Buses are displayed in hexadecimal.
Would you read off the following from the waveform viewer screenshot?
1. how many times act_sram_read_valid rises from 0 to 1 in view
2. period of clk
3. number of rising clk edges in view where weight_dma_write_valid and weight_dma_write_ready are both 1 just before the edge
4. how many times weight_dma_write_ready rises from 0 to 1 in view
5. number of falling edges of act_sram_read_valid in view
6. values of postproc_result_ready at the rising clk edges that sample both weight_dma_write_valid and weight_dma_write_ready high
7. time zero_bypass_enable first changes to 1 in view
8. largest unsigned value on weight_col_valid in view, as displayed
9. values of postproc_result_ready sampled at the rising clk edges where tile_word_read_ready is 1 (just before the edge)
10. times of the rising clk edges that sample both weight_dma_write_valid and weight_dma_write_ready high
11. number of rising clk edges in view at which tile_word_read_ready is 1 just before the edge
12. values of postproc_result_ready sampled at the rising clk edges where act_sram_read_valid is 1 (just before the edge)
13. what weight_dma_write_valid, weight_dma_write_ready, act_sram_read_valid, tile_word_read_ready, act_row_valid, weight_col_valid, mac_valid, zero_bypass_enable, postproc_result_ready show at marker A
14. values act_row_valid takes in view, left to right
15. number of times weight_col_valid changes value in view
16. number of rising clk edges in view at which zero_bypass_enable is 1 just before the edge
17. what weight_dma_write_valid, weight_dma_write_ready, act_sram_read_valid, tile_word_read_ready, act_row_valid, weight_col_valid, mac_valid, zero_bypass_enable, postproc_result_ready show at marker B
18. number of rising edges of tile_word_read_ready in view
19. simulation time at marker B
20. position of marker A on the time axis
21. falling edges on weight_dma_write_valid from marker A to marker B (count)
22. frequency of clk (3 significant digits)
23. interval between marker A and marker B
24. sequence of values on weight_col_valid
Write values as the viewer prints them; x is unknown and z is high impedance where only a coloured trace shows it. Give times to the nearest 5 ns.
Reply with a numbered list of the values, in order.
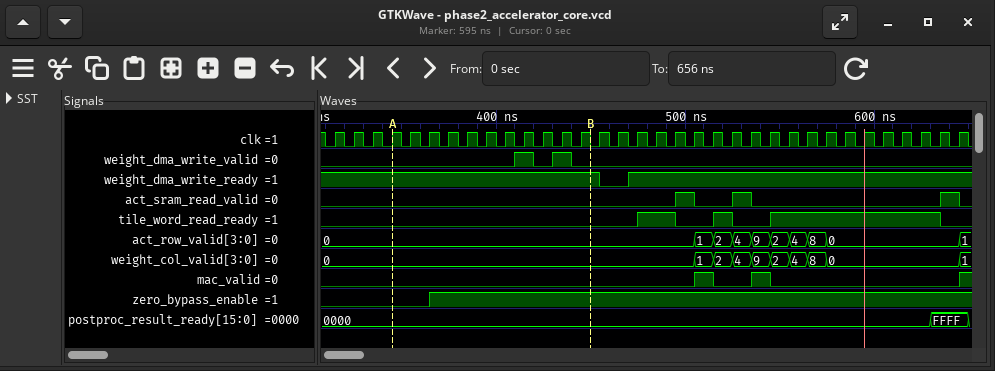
1. 3
2. 10 ns
3. 2
4. 1
5. 3
6. 0000, 0000
7. 365 ns
8. 9
9. 0000, 0000, 0000, 0000, 0000, 0000, 0000, 0000, 0000, 0000, 0000, FFFF
10. 415 ns, 435 ns
11. 12
12. 0000, 0000, FFFF
13. weight_dma_write_valid=0, weight_dma_write_ready=1, act_sram_read_valid=0, tile_word_read_ready=0, act_row_valid=0, weight_col_valid=0, mac_valid=0, zero_bypass_enable=0, postproc_result_ready=0000
14. 0, 1, 2, 4, 9, 2, 4, 8, 0, 1
15. 9
16. 28
17. weight_dma_write_valid=0, weight_dma_write_ready=1, act_sram_read_valid=0, tile_word_read_ready=0, act_row_valid=0, weight_col_valid=0, mac_valid=0, zero_bypass_enable=1, postproc_result_ready=0000
18. 3
19. 450 ns
20. 345 ns
21. 2
22. 100 MHz
23. 105 ns
24. 0, 1, 2, 4, 9, 2, 4, 8, 0, 1
